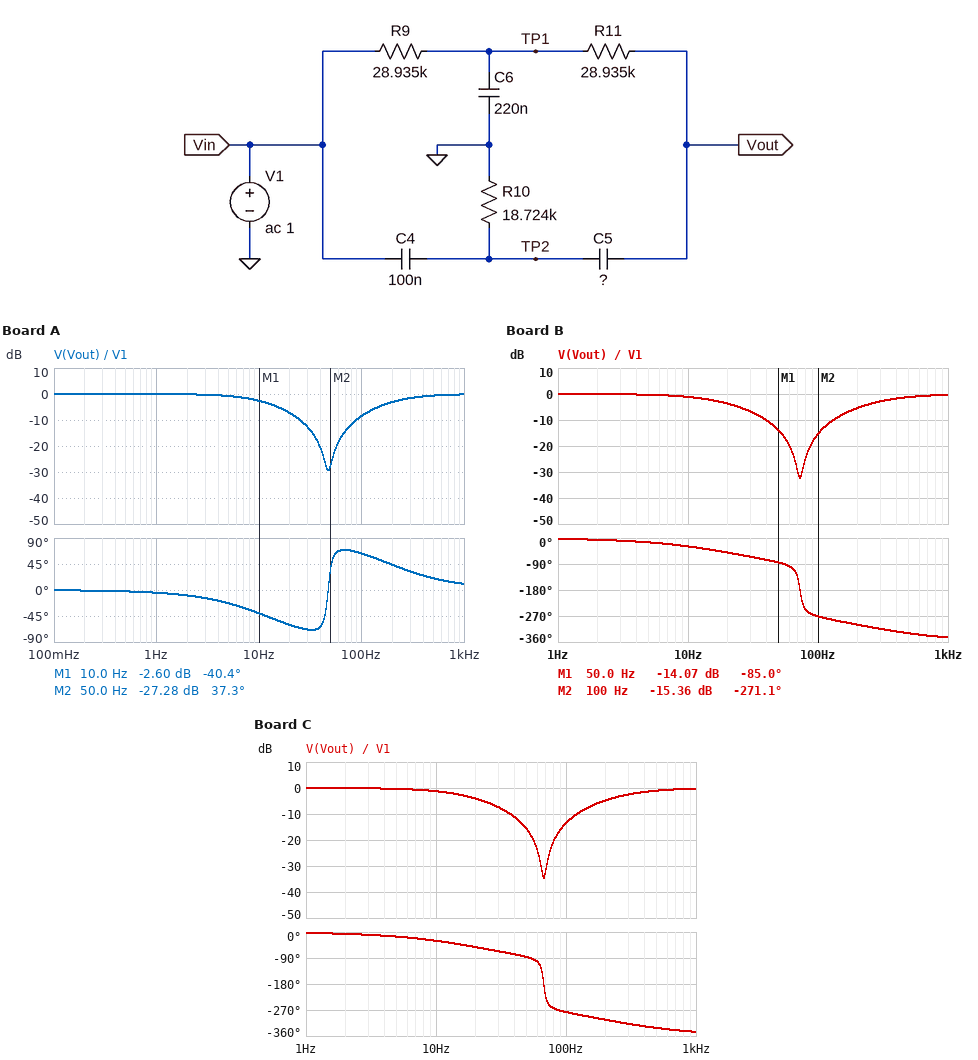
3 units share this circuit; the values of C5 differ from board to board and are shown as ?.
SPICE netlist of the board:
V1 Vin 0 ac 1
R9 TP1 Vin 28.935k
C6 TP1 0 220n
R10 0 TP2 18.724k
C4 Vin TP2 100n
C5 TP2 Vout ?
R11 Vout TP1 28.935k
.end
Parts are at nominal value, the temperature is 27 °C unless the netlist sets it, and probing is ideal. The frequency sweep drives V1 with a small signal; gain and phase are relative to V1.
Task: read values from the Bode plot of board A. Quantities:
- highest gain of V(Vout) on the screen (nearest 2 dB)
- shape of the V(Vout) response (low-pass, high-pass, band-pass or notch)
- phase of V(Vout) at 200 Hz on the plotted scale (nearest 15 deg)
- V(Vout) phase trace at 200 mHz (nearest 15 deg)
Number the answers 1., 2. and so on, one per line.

1. 0 dB
2. notch
3. 45 deg
4. 0 deg
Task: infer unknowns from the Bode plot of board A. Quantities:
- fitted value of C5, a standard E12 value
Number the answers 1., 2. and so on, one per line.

1. 120 nF
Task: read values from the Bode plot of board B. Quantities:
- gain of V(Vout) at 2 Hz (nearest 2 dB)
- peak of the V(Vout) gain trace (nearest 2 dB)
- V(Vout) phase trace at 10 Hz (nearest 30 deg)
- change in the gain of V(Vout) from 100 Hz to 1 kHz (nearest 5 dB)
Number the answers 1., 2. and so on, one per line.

1. 0 dB
2. 0 dB
3. -30 deg
4. 15 dB
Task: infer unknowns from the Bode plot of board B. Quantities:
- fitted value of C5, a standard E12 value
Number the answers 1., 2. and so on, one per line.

1. 39 nF
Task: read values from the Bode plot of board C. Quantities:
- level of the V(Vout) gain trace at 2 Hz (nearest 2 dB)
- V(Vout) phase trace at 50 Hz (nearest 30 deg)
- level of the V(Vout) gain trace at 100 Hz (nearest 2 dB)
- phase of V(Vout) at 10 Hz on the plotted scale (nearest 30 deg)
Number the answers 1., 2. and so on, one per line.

1. 0 dB
2. -90 deg
3. -14 dB
4. -30 deg
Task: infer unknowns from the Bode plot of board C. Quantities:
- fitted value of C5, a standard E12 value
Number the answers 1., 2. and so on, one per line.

1. 47 nF
